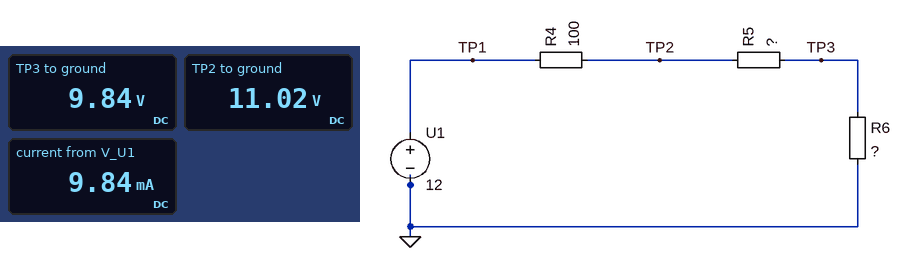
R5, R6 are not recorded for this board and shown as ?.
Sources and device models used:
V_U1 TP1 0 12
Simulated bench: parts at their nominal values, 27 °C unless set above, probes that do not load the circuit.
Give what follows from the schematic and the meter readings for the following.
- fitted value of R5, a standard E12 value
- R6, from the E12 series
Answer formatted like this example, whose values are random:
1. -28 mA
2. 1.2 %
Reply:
1. 120 Ω
2. 1 kΩ
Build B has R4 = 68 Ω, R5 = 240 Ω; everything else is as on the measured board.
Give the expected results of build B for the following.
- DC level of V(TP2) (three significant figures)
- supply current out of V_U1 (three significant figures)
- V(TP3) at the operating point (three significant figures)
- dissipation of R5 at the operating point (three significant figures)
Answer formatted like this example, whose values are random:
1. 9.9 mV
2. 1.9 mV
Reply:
1. 11.4 V
2. 9.17 mA
3. 9.17 V
4. 20.2 mW
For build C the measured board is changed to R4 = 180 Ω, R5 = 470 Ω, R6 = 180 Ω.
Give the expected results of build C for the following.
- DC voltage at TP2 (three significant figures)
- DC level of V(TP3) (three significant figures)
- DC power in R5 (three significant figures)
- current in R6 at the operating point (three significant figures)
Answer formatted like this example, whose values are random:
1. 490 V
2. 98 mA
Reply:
1. 9.40 V
2. 2.60 V
3. 98.2 mW
4. 14.5 mA
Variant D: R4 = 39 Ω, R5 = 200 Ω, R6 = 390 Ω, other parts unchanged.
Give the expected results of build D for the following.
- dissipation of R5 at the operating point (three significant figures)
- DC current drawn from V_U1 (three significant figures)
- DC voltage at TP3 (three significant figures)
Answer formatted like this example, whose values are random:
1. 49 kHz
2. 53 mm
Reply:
1. 72.8 mW
2. 19.1 mA
3. 7.44 V
